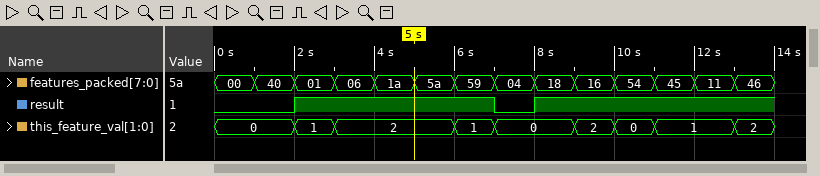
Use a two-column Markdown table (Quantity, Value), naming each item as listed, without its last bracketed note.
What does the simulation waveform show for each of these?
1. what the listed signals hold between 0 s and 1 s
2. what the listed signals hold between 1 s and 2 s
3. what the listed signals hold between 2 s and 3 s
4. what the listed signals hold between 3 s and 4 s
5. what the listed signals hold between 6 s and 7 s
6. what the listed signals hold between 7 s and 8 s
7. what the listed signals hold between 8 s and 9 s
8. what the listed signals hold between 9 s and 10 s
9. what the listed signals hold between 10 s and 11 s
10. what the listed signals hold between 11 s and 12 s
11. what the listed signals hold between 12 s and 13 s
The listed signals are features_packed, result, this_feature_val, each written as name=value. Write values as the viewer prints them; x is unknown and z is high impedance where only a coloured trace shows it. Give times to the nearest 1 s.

| Quantity | Value |
|---|---|
| what the listed signals hold between 0 s and 1 s | features_packed=00, result=0, this_feature_val=0 |
| what the listed signals hold between 1 s and 2 s | features_packed=40, result=0, this_feature_val=0 |
| what the listed signals hold between 2 s and 3 s | features_packed=01, result=1, this_feature_val=1 |
| what the listed signals hold between 3 s and 4 s | features_packed=06, result=1, this_feature_val=2 |
| what the listed signals hold between 6 s and 7 s | features_packed=59, result=1, this_feature_val=1 |
| what the listed signals hold between 7 s and 8 s | features_packed=04, result=0, this_feature_val=0 |
| what the listed signals hold between 8 s and 9 s | features_packed=18, result=1, this_feature_val=0 |
| what the listed signals hold between 9 s and 10 s | features_packed=16, result=1, this_feature_val=2 |
| what the listed signals hold between 10 s and 11 s | features_packed=54, result=1, this_feature_val=0 |
| what the listed signals hold between 11 s and 12 s | features_packed=45, result=1, this_feature_val=1 |
| what the listed signals hold between 12 s and 13 s | features_packed=11, result=1, this_feature_val=1 |
